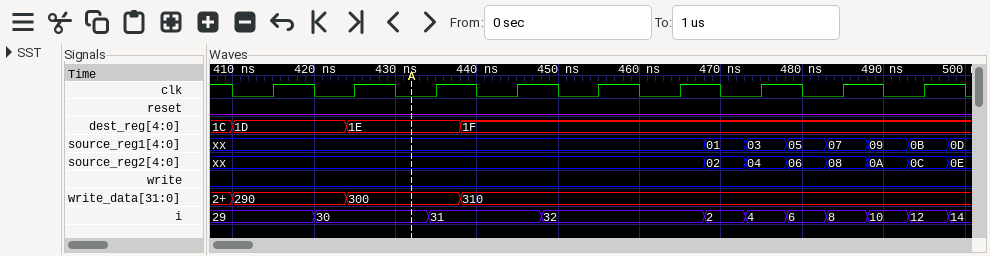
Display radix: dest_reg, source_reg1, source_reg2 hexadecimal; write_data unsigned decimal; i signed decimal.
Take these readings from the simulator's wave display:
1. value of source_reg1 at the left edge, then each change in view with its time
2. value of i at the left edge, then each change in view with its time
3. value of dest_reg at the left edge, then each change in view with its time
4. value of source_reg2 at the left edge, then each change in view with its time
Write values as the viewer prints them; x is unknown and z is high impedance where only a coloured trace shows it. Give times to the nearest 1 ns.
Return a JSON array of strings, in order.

["xx, 01 at 468 ns, 03 at 473 ns, 05 at 478 ns, 07 at 483 ns, 09 at 488 ns, 0B at 493 ns, 0D at 498 ns", "29, 30 at 420 ns, 31 at 434 ns, 32 at 448 ns, 2 at 468 ns, 4 at 473 ns, 6 at 478 ns, 8 at 483 ns, 10 at 488 ns, 12 at 493 ns, 14 at 498 ns", "1C, 1D at 410 ns, 1E at 424 ns, 1F at 438 ns", "xx, 02 at 468 ns, 04 at 473 ns, 06 at 478 ns, 08 at 483 ns, 0A at 488 ns, 0C at 493 ns, 0E at 498 ns"]
